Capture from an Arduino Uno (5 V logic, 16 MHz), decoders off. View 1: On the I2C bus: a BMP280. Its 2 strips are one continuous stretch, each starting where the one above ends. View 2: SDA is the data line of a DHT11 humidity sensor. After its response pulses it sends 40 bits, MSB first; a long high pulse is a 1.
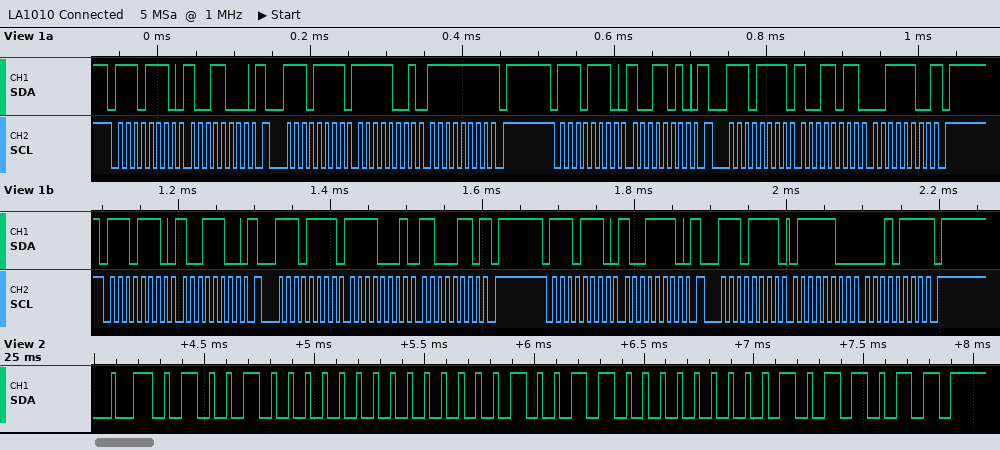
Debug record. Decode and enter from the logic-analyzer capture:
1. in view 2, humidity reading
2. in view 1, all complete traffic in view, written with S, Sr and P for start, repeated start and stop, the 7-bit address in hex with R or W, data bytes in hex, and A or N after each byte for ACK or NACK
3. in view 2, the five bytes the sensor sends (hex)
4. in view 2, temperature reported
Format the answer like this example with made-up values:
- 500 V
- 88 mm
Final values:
- 72 %
- S 77W A 98 A Sr 77R A F9 A FF N P S 77W A 9A A Sr 77R A 9B A 3C N P S 77W A 9C A Sr 77R A F1 A C6 N P S 77W A 9E A Sr 77R A 7C A 17 N P
- 48 00 13 00 5B
- 19.0 °C
